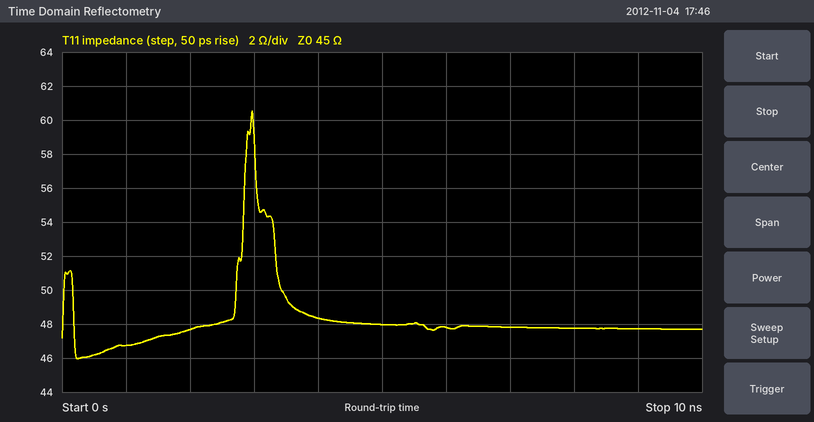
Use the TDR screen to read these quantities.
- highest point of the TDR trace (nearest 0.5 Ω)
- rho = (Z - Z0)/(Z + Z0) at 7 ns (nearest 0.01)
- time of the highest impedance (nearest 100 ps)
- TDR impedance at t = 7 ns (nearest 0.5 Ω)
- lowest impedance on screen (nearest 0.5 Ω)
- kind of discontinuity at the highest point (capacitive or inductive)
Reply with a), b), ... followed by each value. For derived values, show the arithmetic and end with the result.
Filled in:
a) 60.5 Ω
b) (48 − 45)/(48 + 45) ≈ +0.03
c) 3.0 ns
d) 48.0 Ω
e) 46.0 Ω
f) inductive
